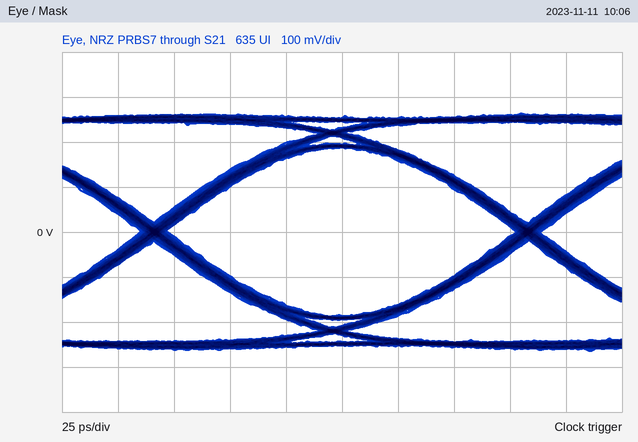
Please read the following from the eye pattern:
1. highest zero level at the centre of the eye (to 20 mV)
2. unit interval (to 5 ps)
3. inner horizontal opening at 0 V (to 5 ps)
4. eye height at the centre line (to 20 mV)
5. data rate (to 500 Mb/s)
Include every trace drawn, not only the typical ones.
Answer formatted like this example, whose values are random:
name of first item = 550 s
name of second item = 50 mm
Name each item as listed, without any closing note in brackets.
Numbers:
highest zero level at the centre of the eye = -180 mV
unit interval = 165 ps
inner horizontal opening at 0 V = 155 ps
eye height at the centre line = 380 mV
data rate = 6.0 Gb/s
